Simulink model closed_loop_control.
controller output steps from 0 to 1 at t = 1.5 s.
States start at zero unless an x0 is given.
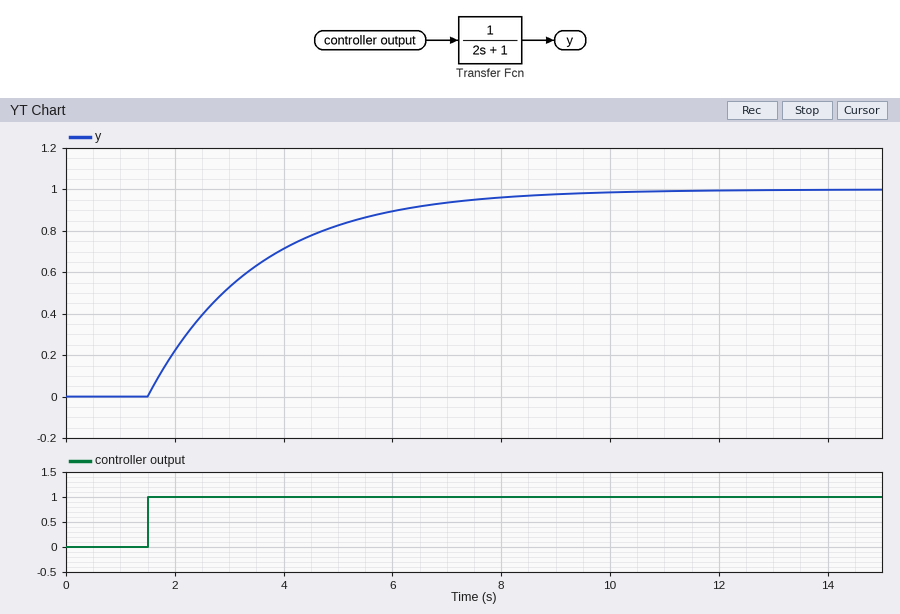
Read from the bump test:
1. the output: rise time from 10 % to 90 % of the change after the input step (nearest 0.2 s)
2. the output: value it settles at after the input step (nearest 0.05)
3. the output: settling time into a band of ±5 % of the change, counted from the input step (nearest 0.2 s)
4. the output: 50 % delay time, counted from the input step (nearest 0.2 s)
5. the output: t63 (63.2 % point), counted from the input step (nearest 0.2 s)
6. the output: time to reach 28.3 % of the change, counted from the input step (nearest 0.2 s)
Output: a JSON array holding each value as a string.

["4.4 s", "1.00", "6.0 s", "1.4 s", "2.0 s", "0.6 s"]
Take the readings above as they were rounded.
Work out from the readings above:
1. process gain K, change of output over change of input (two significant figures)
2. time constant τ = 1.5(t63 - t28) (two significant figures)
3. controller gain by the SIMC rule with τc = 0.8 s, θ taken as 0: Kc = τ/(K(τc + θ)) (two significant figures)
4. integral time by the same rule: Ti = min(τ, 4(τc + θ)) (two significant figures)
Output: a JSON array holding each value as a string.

["1.0", "2.1 s", "2.6", "2.1 s"]
